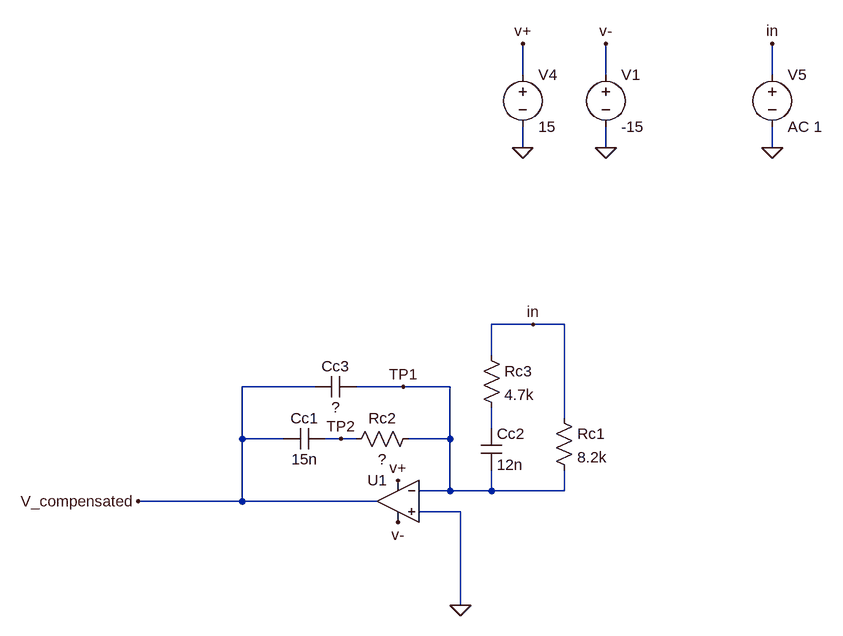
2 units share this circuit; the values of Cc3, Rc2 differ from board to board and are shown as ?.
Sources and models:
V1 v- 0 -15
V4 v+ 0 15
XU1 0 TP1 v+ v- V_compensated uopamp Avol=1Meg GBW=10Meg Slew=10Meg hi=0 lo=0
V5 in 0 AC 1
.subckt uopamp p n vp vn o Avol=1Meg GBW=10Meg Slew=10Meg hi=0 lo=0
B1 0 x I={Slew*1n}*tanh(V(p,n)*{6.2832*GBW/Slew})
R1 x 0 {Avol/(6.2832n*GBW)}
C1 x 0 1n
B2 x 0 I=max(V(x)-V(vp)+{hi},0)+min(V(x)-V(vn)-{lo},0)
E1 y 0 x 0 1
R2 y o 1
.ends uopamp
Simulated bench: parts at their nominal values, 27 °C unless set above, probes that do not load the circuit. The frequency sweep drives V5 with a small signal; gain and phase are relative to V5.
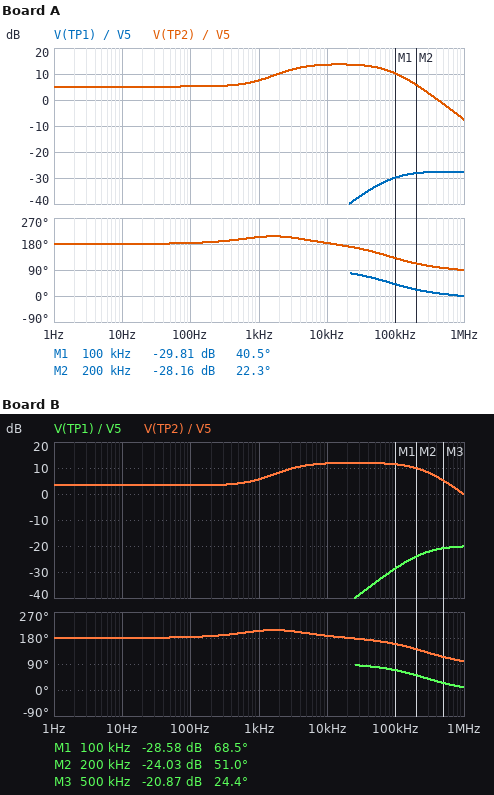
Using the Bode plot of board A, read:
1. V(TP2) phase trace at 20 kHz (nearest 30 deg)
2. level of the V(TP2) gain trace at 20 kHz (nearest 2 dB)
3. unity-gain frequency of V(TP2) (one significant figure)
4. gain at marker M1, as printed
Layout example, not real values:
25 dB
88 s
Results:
180 deg
14 dB
400 kHz
-29.81 dB
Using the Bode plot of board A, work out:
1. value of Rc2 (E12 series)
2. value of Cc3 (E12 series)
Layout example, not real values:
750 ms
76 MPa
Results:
15 kΩ
120 pF
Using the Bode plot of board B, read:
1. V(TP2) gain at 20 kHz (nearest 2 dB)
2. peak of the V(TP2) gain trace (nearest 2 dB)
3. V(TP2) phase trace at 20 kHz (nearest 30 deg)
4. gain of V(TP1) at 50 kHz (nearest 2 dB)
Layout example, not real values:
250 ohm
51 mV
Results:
12 dB
12 dB
180 deg
-34 dB
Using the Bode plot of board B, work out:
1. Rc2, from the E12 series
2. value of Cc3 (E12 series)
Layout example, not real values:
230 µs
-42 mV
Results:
12 kΩ
47 pF
